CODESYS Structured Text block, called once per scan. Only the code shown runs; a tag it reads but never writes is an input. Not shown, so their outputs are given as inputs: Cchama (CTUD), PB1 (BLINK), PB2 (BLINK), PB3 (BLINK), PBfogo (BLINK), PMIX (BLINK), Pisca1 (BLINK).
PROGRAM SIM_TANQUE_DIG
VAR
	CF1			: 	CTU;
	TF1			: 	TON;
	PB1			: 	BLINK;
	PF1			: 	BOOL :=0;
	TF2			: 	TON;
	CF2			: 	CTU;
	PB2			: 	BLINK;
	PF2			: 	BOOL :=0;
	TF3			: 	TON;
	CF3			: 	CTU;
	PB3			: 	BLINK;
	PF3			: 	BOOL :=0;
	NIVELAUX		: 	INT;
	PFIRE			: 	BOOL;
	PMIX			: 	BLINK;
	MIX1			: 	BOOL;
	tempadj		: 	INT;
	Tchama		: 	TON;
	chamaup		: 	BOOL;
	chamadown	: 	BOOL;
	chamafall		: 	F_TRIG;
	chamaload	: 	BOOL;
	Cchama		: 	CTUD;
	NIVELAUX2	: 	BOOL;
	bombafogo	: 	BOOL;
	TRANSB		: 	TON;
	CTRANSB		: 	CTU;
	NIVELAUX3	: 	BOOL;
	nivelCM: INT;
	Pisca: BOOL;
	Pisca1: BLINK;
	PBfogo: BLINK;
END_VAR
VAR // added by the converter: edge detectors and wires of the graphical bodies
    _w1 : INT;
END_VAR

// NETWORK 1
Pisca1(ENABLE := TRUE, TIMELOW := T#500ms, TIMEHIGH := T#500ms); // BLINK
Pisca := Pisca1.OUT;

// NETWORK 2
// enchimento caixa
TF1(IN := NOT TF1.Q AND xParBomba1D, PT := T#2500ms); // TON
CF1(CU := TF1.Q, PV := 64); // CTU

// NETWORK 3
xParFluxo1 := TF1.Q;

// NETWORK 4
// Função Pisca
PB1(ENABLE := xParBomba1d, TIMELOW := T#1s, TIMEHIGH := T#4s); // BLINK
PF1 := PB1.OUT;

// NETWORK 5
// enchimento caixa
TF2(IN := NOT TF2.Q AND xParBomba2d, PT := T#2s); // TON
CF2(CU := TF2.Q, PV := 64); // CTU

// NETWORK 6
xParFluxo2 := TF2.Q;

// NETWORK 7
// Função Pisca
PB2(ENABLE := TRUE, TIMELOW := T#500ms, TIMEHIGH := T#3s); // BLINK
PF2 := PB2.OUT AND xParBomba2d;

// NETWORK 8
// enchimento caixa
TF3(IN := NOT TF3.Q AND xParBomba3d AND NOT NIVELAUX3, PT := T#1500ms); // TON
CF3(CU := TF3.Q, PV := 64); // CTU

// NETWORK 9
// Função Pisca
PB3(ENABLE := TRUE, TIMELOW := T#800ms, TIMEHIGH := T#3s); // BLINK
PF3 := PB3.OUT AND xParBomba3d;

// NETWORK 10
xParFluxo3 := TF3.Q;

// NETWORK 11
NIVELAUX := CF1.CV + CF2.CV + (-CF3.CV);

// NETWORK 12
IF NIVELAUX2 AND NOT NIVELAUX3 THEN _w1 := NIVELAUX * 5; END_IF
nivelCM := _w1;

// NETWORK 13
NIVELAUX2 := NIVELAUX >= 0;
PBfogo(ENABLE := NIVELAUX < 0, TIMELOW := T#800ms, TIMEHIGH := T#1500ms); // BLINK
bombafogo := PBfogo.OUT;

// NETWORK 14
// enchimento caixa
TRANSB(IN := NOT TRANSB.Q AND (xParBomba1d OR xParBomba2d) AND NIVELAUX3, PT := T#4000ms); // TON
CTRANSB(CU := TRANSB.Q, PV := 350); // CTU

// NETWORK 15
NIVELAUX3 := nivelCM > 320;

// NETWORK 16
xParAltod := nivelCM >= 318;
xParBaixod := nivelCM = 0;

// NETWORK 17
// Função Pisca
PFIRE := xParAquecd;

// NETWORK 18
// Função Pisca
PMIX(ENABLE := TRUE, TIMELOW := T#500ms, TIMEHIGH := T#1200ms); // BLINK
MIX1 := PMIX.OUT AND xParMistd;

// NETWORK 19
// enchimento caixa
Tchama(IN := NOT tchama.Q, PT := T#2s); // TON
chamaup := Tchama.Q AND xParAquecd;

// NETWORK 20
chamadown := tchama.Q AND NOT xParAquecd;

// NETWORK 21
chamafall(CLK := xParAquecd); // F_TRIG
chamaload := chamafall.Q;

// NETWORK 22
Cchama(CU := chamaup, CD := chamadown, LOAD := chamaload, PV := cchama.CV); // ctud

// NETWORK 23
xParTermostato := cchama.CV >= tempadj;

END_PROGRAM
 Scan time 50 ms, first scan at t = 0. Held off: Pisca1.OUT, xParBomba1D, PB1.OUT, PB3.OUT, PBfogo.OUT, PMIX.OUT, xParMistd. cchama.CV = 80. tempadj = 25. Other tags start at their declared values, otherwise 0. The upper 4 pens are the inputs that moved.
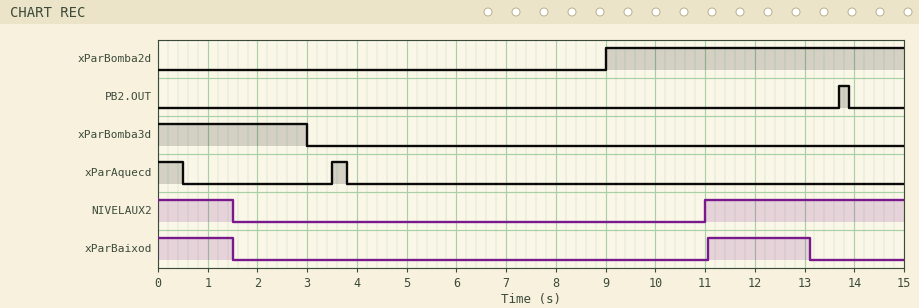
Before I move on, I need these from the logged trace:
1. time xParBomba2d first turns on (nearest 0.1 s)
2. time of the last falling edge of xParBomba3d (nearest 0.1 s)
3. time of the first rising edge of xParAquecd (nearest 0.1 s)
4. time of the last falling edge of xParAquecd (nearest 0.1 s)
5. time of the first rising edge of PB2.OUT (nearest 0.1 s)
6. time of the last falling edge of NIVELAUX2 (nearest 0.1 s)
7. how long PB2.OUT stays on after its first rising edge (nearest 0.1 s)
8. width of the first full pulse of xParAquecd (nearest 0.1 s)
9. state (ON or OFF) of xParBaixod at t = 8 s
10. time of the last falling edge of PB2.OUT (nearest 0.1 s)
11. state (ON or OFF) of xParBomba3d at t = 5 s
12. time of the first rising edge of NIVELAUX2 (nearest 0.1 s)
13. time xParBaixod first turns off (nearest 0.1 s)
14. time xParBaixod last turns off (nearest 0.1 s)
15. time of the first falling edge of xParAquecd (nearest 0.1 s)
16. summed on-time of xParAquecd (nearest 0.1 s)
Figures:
9.0 s
3.0 s
3.5 s
3.8 s
13.7 s
1.5 s
0.2 s
0.3 s
OFF
13.9 s
OFF
11.0 s
1.5 s
13.1 s
0.5 s
0.8 s
